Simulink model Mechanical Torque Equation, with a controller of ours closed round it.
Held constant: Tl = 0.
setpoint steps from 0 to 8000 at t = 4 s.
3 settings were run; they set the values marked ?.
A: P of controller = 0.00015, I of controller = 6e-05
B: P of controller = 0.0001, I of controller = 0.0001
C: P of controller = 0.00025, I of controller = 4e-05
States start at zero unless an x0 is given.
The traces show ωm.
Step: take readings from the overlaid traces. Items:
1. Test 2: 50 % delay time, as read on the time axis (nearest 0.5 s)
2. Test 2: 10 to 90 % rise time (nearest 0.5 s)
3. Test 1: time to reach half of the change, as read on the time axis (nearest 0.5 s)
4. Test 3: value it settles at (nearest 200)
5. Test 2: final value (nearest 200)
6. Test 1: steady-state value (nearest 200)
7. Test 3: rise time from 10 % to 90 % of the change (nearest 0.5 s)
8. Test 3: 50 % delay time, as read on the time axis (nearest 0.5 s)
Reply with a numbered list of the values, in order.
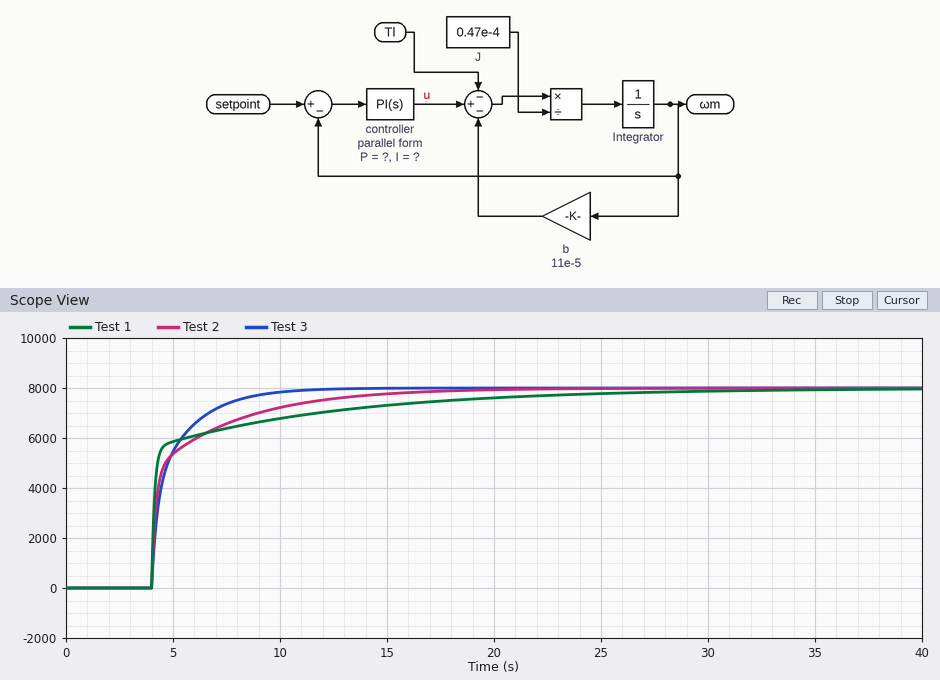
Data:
1. 4.5 s
2. 6.0 s
3. 4.0 s
4. 8000
5. 8000
6. 8000
7. 3.0 s
8. 4.5 s
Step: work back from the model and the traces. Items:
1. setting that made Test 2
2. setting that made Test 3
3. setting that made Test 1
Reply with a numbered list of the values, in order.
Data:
1. A
2. B
3. C
